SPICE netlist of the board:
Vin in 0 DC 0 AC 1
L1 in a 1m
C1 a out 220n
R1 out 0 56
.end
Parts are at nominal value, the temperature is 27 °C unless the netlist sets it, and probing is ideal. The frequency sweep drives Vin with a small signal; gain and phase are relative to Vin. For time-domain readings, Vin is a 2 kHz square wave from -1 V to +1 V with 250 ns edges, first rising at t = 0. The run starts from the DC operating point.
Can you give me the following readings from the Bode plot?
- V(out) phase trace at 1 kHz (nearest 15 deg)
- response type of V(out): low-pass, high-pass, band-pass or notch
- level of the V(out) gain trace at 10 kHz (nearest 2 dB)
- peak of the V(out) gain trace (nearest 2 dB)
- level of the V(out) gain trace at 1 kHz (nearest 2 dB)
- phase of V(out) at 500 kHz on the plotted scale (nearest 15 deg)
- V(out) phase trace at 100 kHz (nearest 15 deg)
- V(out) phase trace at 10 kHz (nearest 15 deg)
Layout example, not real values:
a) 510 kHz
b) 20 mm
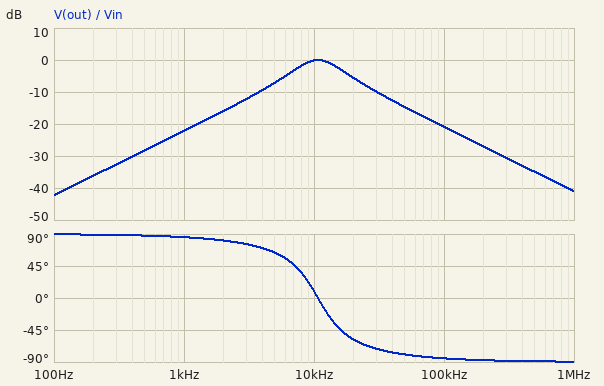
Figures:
a) 90 deg
b) band-pass
c) 0 dB
d) 0 dB
e) -22 dB
f) -90 deg
g) -90 deg
h) 15 deg
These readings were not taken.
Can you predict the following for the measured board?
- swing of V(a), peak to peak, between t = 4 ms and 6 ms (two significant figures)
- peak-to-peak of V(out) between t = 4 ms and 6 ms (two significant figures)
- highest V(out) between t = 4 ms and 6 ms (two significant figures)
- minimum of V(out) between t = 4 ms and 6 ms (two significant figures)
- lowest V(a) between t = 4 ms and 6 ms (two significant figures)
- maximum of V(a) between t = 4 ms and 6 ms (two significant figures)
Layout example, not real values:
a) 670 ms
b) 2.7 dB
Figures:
a) 3.4 V
b) 2.0 V
c) 990 mV
d) -990 mV
e) -1.7 V
f) 1.7 V
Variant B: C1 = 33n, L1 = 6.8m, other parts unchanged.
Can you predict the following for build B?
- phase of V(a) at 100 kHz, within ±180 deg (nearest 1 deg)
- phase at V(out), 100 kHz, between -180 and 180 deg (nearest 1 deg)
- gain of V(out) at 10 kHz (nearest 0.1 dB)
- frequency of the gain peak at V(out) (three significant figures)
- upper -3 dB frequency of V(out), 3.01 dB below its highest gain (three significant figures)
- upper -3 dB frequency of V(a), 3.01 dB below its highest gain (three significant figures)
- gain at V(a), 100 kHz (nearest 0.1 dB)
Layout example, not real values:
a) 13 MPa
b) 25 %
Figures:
a) -130 deg
b) -89 deg
c) -2.9 dB
d) 10.6 kHz
e) 11.3 kHz
f) 11.2 kHz
g) -35.1 dB
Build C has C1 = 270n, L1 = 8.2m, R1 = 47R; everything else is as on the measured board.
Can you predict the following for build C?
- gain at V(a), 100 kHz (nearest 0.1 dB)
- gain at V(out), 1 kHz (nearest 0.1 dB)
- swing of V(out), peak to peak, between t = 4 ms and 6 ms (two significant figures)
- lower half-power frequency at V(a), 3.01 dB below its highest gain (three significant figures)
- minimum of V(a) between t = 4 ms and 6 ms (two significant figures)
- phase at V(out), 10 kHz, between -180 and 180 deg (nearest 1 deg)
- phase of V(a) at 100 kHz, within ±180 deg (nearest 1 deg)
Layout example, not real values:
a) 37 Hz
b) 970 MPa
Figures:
a) -40.7 dB
b) -21.2 dB
c) 700 mV
d) 2.83 kHz
e) -2.1 V
f) -84 deg
g) -97 deg
